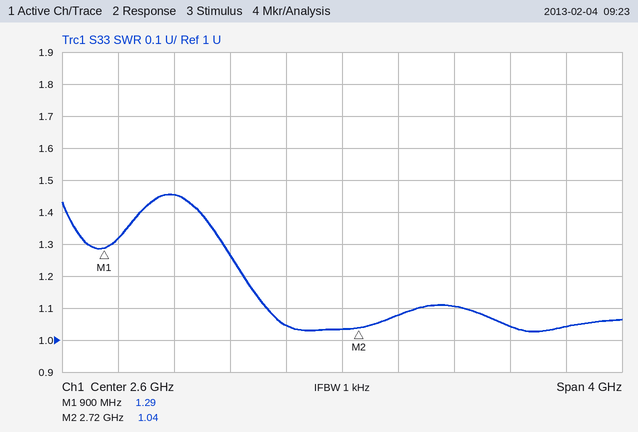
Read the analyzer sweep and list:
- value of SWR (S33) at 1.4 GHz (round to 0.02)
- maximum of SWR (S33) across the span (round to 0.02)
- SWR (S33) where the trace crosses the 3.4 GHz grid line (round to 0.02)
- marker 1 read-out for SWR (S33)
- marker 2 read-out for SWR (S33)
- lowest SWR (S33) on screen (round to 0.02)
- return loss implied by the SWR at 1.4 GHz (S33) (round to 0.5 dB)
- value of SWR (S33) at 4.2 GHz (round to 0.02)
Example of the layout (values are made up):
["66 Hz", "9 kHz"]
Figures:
["1.46", "1.46", "1.10", "1.29", "1.04", "1.02", "14.5 dB", "1.04"]
